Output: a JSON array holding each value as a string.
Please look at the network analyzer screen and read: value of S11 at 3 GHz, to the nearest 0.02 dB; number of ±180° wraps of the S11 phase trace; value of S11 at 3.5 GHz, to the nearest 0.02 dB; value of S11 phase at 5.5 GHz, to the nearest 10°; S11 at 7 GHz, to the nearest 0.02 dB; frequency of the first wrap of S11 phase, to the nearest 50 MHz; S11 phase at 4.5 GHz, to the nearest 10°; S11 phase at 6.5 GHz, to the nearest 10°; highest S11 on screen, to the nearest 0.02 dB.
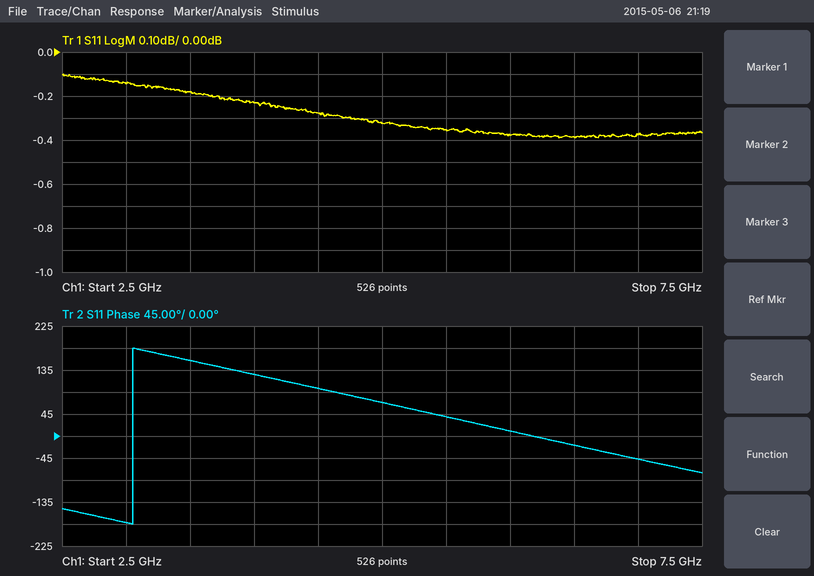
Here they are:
["-0.14 dB", "1", "-0.18 dB", "40°", "-0.38 dB", "3.05 GHz", "100°", "-20°", "-0.10 dB"]
